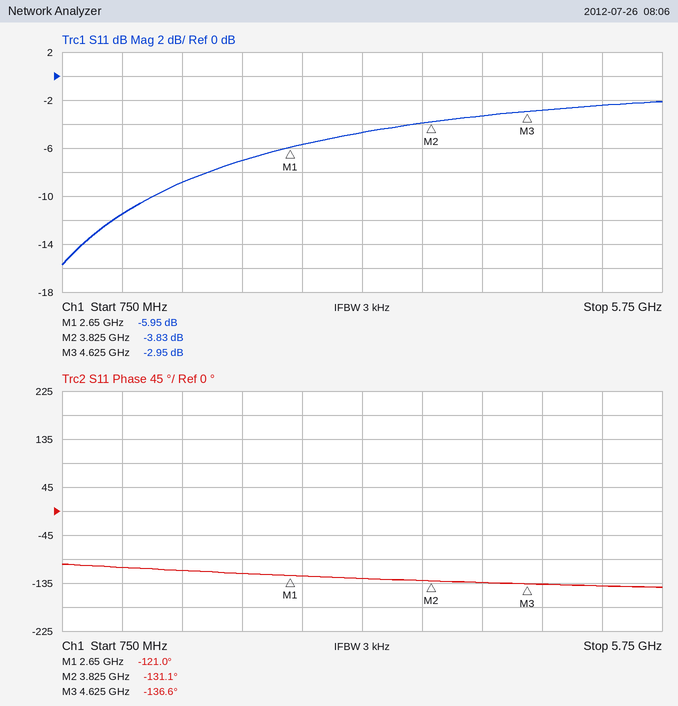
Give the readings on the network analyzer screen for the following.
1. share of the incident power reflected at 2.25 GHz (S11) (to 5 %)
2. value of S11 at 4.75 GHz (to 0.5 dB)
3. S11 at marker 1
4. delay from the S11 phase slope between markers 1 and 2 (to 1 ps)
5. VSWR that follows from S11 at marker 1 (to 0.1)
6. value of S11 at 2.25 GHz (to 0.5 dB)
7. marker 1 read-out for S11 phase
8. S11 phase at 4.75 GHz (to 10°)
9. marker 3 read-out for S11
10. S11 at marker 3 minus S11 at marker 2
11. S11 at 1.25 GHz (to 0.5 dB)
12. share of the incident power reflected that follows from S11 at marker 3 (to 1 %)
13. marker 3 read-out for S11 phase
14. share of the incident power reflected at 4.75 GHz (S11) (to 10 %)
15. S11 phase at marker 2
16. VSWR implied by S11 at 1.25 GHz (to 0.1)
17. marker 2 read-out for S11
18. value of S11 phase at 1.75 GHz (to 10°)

20 %
-3.0 dB
-5.95 dB
24 ps
3.0
-7.0 dB
-121.0°
-140°
-2.95 dB
0.88 dB
-11.5 dB
51 %
-136.6°
50 %
-131.1°
1.7
-3.83 dB
-110°
